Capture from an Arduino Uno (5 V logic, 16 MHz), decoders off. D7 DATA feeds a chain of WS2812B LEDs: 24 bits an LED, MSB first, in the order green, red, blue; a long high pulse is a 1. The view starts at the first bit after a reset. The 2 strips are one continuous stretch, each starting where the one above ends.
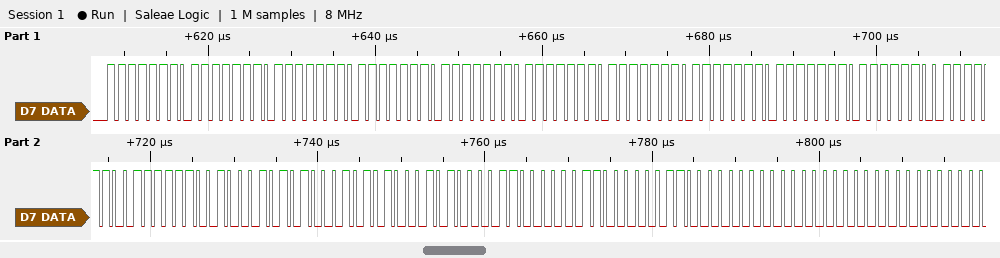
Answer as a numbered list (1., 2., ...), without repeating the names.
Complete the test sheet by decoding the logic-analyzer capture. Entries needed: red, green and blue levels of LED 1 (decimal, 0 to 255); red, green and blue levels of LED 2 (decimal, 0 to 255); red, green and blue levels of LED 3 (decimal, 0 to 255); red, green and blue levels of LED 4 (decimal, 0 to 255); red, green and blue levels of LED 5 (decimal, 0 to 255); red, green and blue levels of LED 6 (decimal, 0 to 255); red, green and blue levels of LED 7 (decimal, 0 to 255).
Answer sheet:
1. 254, 254, 254
2. 254, 254, 254
3. 254, 254, 254
4. 252, 252, 252
5. 138, 138, 138
6. 24, 24, 24
7. 0, 0, 0
